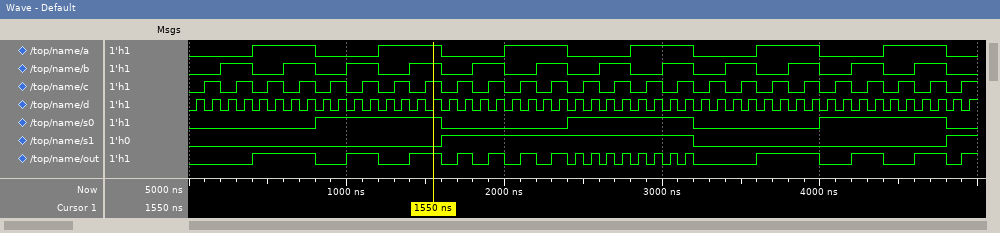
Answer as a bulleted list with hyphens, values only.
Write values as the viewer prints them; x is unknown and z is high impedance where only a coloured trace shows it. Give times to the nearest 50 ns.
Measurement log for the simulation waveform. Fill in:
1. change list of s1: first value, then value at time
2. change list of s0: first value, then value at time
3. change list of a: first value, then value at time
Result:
- 0, 1 at 1600 ns, 0 at 3200 ns, 1 at 4800 ns
- 0, 1 at 800 ns, 0 at 1600 ns, 1 at 2400 ns, 0 at 3200 ns, 1 at 4000 ns, 0 at 4800 ns
- 0, 1 at 400 ns, 0 at 800 ns, 1 at 1200 ns, 0 at 1600 ns, 1 at 2000 ns, 0 at 2400 ns, 1 at 2800 ns, 0 at 3200 ns, 1 at 3600 ns, 0 at 4000 ns, 1 at 4400 ns, 0 at 4800 ns
